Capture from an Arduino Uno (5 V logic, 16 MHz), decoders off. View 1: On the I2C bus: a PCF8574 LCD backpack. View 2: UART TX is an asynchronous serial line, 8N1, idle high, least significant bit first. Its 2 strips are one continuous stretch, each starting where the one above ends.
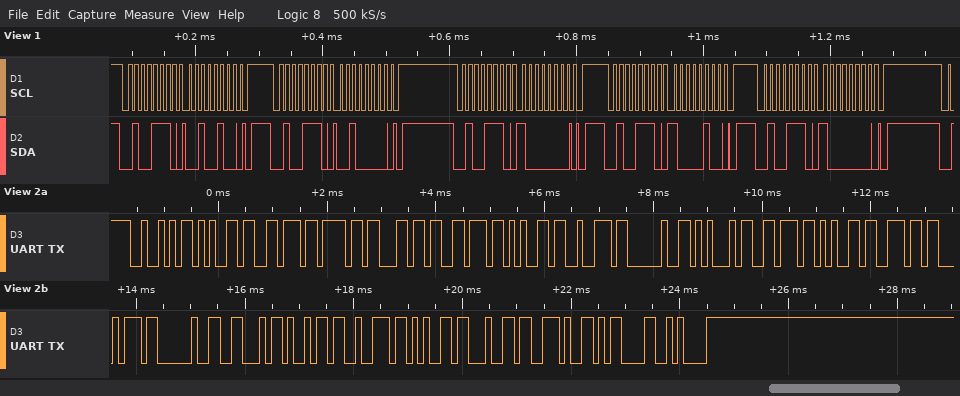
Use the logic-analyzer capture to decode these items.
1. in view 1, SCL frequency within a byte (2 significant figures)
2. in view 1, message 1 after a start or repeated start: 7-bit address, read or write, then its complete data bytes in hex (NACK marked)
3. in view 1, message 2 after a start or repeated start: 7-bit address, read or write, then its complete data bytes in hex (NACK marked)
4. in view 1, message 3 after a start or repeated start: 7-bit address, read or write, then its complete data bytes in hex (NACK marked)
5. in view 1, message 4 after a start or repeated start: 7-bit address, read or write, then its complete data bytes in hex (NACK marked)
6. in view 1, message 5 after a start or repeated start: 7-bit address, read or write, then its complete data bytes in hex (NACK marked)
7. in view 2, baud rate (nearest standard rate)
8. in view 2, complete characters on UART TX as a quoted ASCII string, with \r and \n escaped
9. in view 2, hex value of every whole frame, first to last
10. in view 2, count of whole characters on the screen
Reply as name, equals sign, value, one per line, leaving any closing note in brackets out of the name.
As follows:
in view 1, SCL frequency within a byte = 100 kHz
in view 1, message 1 after a start or repeated start: 7-bit address, read or write, then its complete data bytes in hex = 0x27 write: 24
in view 1, message 2 after a start or repeated start: 7-bit address, read or write, then its complete data bytes in hex = 0x27 write: 20
in view 1, message 3 after a start or repeated start: 7-bit address, read or write, then its complete data bytes in hex = 0x27 write: 80
in view 1, message 4 after a start or repeated start: 7-bit address, read or write, then its complete data bytes in hex = 0x27 write: 84
in view 1, message 5 after a start or repeated start: 7-bit address, read or write, then its complete data bytes in hex = 0x27 write: 80
in view 2, baud rate = 9600 baud
in view 2, complete characters on UART TX as a quoted ASCII string, with \r and \n escaped = "Revolver Event Fired.\r\n"
in view 2, hex value of every whole frame, first to last = 52 65 76 6F 6C 76 65 72 20 45 76 65 6E 74 20 46 69 72 65 64 2E 0D 0A
in view 2, count of whole characters on the screen = 23
